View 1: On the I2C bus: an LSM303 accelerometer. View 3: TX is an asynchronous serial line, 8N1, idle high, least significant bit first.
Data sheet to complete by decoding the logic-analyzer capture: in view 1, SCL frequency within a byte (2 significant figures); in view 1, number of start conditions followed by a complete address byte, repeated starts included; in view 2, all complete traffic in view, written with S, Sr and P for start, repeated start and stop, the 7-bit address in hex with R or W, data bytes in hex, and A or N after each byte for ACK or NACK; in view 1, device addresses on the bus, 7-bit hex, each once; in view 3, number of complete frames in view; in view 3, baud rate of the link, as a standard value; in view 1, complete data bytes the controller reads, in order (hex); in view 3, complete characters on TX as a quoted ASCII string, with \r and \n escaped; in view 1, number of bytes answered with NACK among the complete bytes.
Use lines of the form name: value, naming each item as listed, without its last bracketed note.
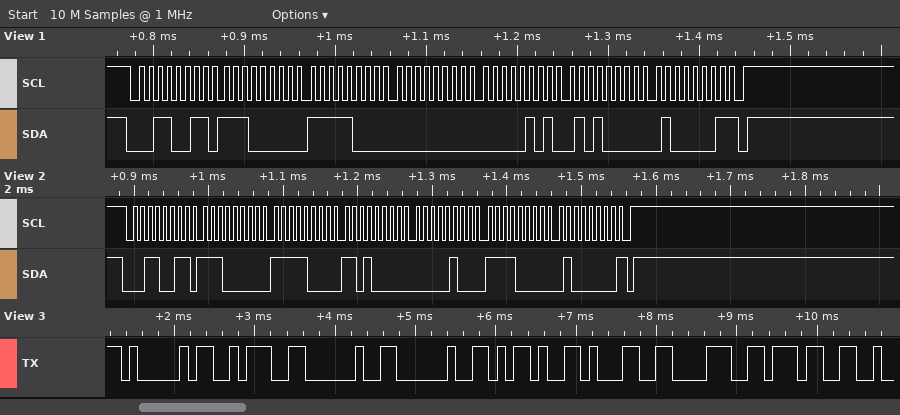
in view 1, SCL frequency within a byte: 100 kHz
in view 1, number of start conditions followed by a complete address byte, repeated starts included: 1
in view 2, all complete traffic in view, written with S, Sr and P for start, repeated start and stop, the 7-bit address in hex with R or W, data bytes in hex, and A or N after each byte for ACK or NACK: S 19R A E0 A F8 A D0 A 04 A F0 A 40 N P
in view 1, device addresses on the bus, 7-bit hex, each once: 0x19
in view 3, number of complete frames in view: 8
in view 3, baud rate of the link, as a standard value: 9600 baud
in view 1, complete data bytes the controller reads, in order: E0 F8 00 05 50 41
in view 3, complete characters on TX as a quoted ASCII string, with \r and \n escaped: "A:  -187"
in view 1, number of bytes answered with NACK among the complete bytes: 1
